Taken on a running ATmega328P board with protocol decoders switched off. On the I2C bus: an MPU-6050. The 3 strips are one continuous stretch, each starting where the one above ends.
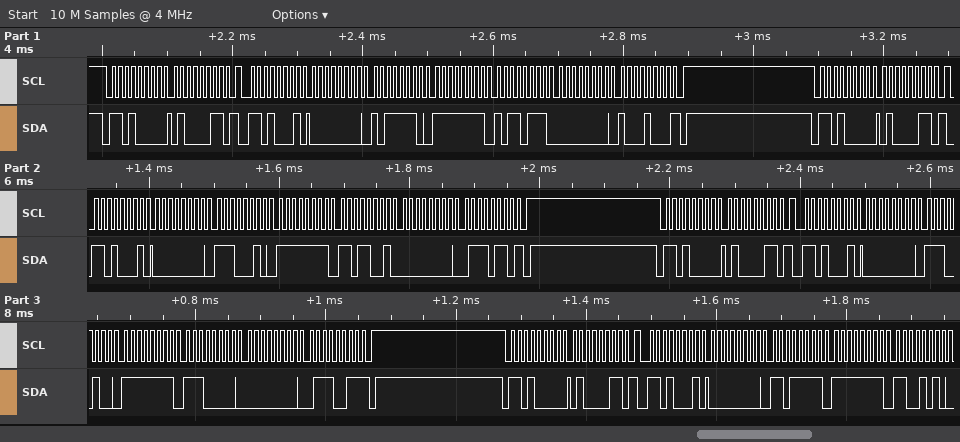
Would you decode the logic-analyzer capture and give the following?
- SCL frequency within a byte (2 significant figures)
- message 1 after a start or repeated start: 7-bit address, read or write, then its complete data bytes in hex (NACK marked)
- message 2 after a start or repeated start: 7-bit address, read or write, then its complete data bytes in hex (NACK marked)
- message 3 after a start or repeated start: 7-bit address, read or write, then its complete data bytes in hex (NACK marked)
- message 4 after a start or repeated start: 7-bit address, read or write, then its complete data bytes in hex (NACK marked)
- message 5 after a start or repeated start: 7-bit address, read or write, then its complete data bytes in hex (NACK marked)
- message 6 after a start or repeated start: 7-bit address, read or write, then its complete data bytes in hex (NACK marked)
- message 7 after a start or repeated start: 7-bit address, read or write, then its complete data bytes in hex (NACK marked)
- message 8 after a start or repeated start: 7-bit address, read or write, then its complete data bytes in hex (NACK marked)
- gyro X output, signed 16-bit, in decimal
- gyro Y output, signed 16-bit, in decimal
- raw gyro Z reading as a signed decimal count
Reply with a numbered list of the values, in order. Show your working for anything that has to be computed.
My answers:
1. 100 kHz
2. 0x68 write: 43
3. 0x68 read: 00 BE FF B7 00 88 NACK
4. 0x68 write: 43
5. 0x68 read: 00 E2 FF D9 00 76 NACK
6. 0x68 write: 43
7. 0x68 read: 00 E4 FF E0 00 73 NACK
8. 0x68 write: 43
9. 0x68 read: 00 DF FF CA
10. 0x00BE = 190
11. 0xFFB7 = -73
12. 0x0088 = 136
